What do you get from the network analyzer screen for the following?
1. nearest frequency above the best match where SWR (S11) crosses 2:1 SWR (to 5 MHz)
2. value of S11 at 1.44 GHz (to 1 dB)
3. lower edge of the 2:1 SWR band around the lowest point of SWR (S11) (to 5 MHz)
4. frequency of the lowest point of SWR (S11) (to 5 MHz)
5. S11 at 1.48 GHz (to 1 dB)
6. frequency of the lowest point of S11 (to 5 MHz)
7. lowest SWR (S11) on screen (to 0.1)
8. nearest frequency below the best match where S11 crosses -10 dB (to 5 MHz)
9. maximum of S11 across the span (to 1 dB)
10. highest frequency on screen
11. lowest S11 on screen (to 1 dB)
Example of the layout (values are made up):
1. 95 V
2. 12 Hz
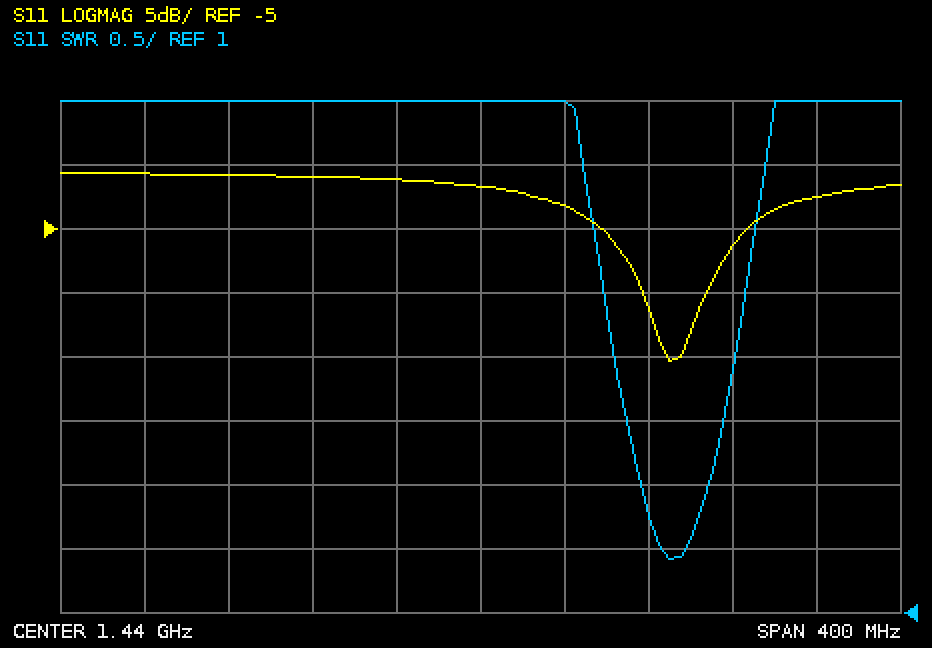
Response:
1. 1.550 GHz
2. -2 dB
3. 1.515 GHz
4. 1.530 GHz
5. -3 dB
6. 1.530 GHz
7. 1.4
8. 1.515 GHz
9. -1 dB
10. 1.64 GHz
11. -15 dB
